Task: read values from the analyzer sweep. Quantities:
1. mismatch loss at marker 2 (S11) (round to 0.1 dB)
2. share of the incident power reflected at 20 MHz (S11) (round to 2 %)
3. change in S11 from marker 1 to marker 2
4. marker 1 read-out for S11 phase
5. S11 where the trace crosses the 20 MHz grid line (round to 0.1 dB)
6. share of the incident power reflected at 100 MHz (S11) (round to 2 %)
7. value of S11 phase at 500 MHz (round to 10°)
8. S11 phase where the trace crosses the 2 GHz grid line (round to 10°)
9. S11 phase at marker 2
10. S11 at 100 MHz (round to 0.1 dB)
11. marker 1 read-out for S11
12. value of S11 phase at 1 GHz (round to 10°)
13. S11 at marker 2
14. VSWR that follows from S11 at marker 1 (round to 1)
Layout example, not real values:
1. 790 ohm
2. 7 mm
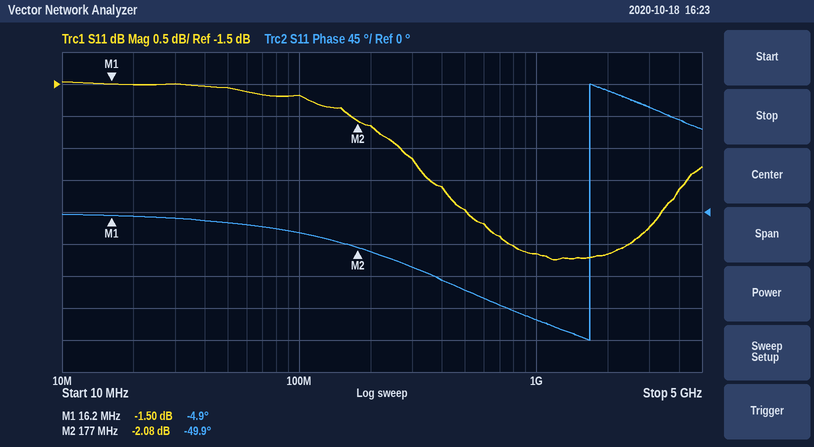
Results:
1. 4.2 dB
2. 70 %
3. -0.58 dB
4. -4.9°
5. -1.5 dB
6. 68 %
7. -110°
8. 170°
9. -49.9°
10. -1.7 dB
11. -1.50 dB
12. -150°
13. -2.08 dB
14. 12
